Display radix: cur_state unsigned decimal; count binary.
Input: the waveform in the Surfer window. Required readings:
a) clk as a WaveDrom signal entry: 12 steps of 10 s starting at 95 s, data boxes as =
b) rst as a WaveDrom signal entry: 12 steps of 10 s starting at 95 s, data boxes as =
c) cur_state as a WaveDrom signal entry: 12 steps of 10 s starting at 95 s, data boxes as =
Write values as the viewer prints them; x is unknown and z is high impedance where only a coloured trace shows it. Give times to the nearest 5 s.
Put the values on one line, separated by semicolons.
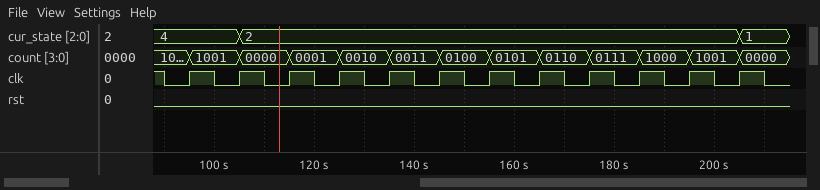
{name: 'clk', wave: 'p...........'}; {name: 'rst', wave: '0...........'}; {name: 'cur_state', wave: '==.........=', data: '4 2 1'}
